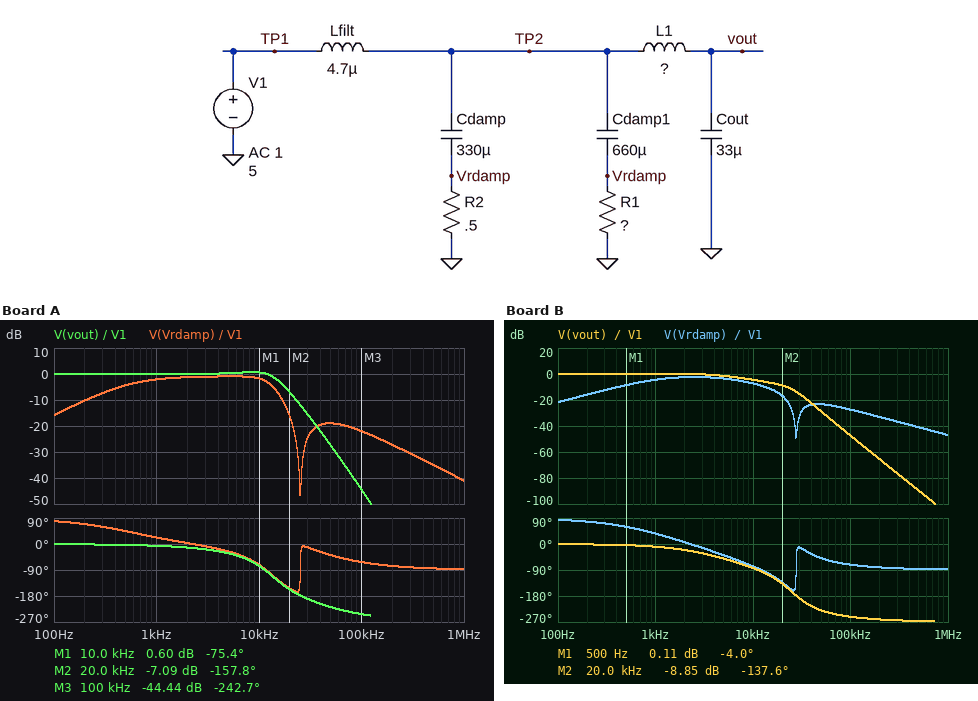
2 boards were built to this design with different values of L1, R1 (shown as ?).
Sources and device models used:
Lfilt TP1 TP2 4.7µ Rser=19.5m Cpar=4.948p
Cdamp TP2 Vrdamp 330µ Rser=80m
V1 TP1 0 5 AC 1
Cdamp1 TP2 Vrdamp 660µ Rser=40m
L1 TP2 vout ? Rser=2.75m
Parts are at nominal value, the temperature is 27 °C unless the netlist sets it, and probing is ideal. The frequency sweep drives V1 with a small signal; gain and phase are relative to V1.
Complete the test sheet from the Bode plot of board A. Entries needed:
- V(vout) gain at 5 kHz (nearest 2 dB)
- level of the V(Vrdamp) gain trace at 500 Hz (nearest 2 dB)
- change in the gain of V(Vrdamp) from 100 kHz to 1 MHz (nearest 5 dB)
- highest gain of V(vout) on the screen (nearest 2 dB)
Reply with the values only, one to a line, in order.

0 dB
-4 dB
-20 dB
0 dB
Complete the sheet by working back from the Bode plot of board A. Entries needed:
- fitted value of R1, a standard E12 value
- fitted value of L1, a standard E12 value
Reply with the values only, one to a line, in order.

0.56 Ω
1.2 µH
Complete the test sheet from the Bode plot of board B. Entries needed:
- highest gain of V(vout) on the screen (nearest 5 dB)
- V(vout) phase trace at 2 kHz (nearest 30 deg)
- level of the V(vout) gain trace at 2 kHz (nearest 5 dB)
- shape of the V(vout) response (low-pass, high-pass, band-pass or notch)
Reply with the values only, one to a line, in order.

0 dB
-30 deg
0 dB
low-pass
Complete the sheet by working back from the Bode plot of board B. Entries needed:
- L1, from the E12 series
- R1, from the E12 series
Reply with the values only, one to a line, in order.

1 µH
0.18 Ω
